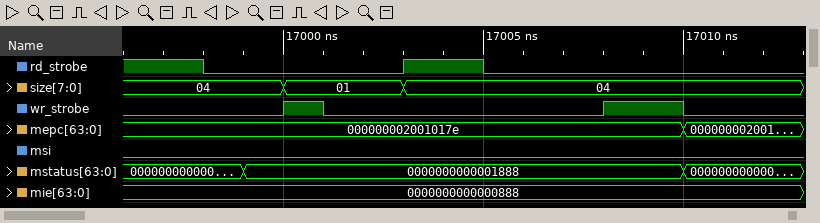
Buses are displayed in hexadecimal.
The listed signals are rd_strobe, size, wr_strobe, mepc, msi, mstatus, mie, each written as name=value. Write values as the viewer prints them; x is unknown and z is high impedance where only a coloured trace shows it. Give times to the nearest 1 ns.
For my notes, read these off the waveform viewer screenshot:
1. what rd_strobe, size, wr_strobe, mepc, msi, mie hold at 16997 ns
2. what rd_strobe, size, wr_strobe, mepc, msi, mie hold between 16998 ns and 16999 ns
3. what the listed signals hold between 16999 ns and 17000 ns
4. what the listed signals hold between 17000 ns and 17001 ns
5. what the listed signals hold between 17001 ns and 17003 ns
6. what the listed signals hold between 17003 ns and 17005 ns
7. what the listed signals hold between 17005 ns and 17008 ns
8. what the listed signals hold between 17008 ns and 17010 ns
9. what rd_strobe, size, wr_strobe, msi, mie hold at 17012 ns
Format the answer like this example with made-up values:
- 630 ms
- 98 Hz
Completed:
- rd_strobe=1, size=04, wr_strobe=0, mepc=000000002001017e, msi=0, mie=0000000000000888
- rd_strobe=0, size=04, wr_strobe=0, mepc=000000002001017e, msi=0, mie=0000000000000888
- rd_strobe=0, size=04, wr_strobe=0, mepc=000000002001017e, msi=0, mstatus=0000000000001888, mie=0000000000000888
- rd_strobe=0, size=01, wr_strobe=1, mepc=000000002001017e, msi=0, mstatus=0000000000001888, mie=0000000000000888
- rd_strobe=0, size=01, wr_strobe=0, mepc=000000002001017e, msi=0, mstatus=0000000000001888, mie=0000000000000888
- rd_strobe=1, size=04, wr_strobe=0, mepc=000000002001017e, msi=0, mstatus=0000000000001888, mie=0000000000000888
- rd_strobe=0, size=04, wr_strobe=0, mepc=000000002001017e, msi=0, mstatus=0000000000001888, mie=0000000000000888
- rd_strobe=0, size=04, wr_strobe=1, mepc=000000002001017e, msi=0, mstatus=0000000000001888, mie=0000000000000888
- rd_strobe=0, size=04, wr_strobe=0, msi=0, mie=0000000000000888
